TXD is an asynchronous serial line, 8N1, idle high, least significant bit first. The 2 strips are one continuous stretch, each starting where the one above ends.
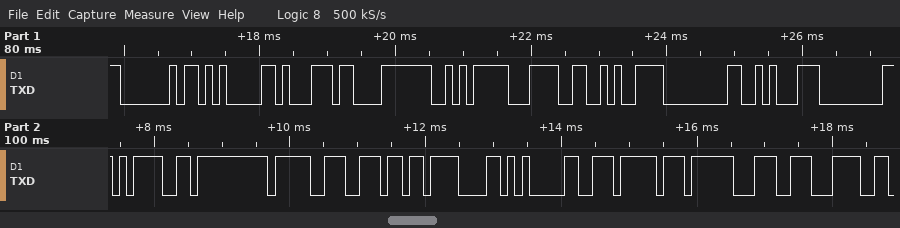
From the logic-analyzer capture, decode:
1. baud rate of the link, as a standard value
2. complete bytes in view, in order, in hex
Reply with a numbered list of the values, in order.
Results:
1. 9600 baud
2. 0x40 0x05 0x71 0xF8 0xEA 0x3C 0xCA 0x00 0x8A 0x00 0x3D 0xFF 0x9F 0x6E 0x0F 0x05 0xEE 0xF7 0x9C 0x3C
